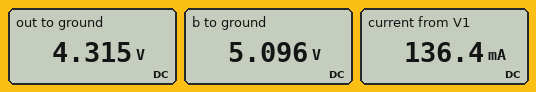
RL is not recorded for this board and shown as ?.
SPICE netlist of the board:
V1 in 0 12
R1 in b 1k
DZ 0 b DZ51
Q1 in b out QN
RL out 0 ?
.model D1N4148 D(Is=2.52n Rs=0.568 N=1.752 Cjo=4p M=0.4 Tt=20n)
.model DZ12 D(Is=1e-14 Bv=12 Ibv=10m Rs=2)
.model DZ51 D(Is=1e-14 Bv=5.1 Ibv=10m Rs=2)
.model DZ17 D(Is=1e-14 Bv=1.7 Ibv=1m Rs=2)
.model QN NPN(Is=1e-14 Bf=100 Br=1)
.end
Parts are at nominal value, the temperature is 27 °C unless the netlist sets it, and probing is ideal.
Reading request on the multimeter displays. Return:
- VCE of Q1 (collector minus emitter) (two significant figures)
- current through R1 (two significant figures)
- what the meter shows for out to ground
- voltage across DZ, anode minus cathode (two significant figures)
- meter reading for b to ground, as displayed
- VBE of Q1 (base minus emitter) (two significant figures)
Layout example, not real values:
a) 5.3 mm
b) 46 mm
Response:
a) 7.7 V
b) 6.9 mA
c) 4.315 V
d) -5.1 V
e) 5.096 V
f) 780 mV
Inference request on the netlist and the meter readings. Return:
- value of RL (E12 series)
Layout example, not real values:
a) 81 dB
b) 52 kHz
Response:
a) 33 Ω
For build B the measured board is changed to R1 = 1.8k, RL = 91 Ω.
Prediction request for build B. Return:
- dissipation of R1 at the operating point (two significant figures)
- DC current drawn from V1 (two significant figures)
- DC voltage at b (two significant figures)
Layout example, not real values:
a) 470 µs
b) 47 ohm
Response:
a) 27 mW
b) 51 mA
c) 5.1 V
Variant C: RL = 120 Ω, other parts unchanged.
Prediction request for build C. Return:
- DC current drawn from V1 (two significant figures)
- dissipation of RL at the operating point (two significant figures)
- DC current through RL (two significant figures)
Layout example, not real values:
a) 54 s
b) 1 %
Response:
a) 43 mA
b) 160 mW
c) 36 mA
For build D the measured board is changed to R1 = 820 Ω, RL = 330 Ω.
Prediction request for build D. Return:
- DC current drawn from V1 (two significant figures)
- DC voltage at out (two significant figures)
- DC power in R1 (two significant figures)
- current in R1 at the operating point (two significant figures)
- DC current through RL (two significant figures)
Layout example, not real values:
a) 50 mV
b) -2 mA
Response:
a) 22 mA
b) 4.4 V
c) 58 mW
d) 8.4 mA
e) 13 mA
